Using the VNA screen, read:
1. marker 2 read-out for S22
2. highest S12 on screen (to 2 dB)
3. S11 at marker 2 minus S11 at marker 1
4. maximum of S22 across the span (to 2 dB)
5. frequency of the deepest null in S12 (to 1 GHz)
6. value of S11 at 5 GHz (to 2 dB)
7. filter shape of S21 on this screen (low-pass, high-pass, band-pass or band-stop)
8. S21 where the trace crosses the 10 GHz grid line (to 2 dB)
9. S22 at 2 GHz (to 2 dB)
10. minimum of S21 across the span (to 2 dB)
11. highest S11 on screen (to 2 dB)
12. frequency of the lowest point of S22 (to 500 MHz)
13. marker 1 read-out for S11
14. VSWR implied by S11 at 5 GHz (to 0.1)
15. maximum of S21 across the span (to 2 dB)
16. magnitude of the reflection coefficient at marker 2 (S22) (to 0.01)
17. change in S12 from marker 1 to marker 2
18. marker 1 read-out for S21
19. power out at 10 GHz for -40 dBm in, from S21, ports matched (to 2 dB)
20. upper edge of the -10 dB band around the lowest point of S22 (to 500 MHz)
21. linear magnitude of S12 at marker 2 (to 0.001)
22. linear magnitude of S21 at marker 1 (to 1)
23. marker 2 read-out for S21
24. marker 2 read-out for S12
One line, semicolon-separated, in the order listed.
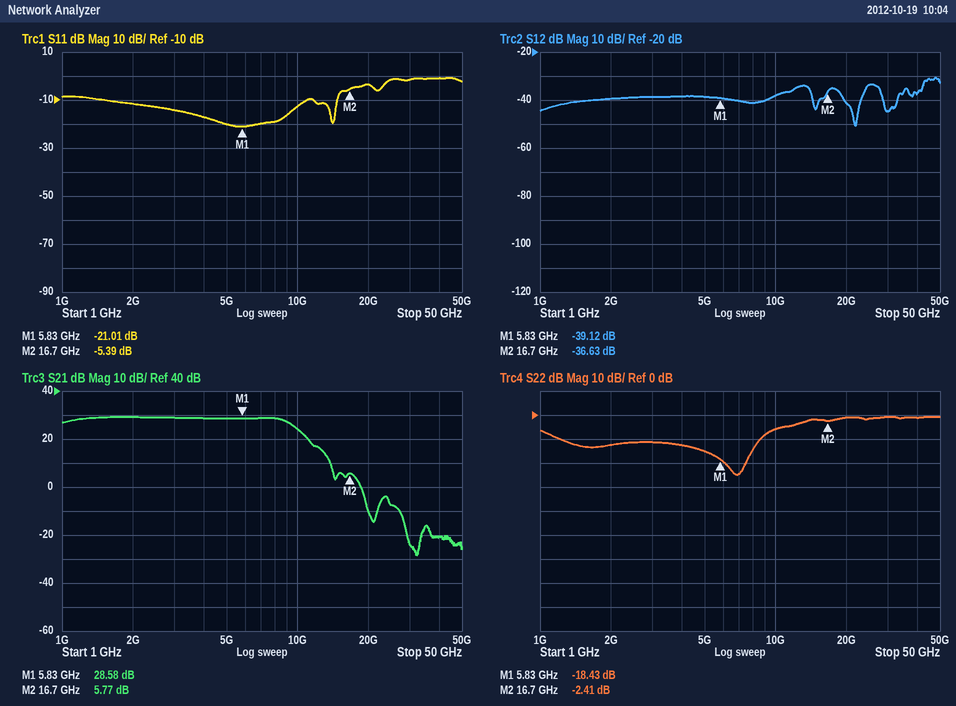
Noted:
-2.41 dB; -30 dB; 15.62 dB; 0 dB; 22 GHz; -20 dB; low-pass; 24 dB; -12 dB; -28 dB; 0 dB; 7.0 GHz; -21.01 dB; 1.2; 30 dB; 0.76; 2.49 dB; 28.58 dB; -16 dBm; 8.5 GHz; 0.015; 27; 5.77 dB; -36.63 dB
